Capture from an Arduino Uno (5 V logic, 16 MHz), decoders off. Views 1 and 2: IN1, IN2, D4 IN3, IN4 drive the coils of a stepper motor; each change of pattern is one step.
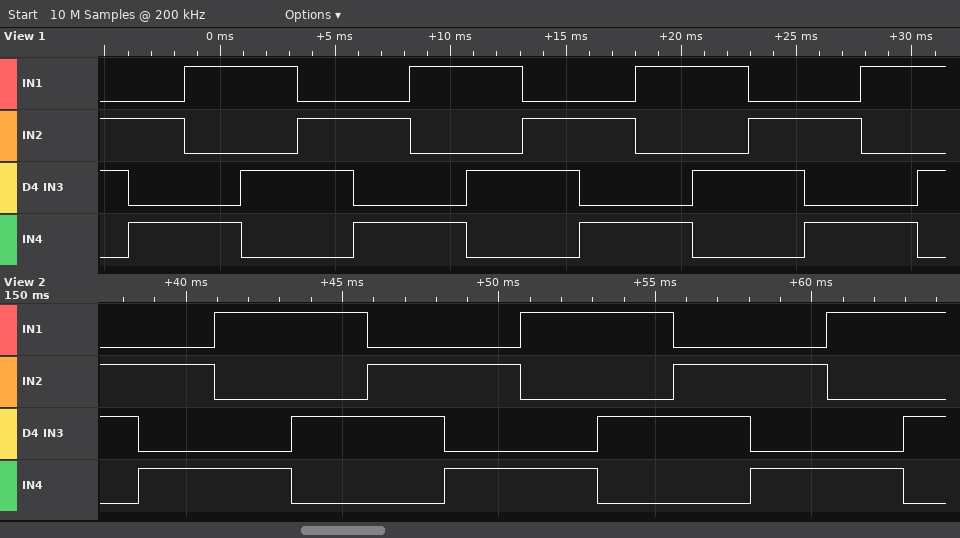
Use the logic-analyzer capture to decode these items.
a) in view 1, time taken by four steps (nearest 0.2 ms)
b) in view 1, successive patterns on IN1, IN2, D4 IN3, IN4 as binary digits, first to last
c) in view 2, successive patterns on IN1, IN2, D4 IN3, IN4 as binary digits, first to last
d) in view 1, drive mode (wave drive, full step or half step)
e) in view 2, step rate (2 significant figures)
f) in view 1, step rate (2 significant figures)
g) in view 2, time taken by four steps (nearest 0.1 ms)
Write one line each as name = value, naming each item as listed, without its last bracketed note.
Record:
in view 1, time taken by four steps = 9.8 ms
in view 1, successive patterns on IN1, IN2, D4 IN3, IN4 as binary digits, first to last = 0110 0101 1001 1010 0110 0101 1001 1010 0110 0101 1001 1010 0110 0101 1001 1010
in view 2, successive patterns on IN1, IN2, D4 IN3, IN4 as binary digits, first to last = 0110 0101 1001 1010 0110 0101 1001 1010 0110 0101 1001 1010
in view 1, drive mode = full step
in view 2, step rate = 410 steps/s
in view 1, step rate = 410 steps/s
in view 2, time taken by four steps = 9.8 ms
